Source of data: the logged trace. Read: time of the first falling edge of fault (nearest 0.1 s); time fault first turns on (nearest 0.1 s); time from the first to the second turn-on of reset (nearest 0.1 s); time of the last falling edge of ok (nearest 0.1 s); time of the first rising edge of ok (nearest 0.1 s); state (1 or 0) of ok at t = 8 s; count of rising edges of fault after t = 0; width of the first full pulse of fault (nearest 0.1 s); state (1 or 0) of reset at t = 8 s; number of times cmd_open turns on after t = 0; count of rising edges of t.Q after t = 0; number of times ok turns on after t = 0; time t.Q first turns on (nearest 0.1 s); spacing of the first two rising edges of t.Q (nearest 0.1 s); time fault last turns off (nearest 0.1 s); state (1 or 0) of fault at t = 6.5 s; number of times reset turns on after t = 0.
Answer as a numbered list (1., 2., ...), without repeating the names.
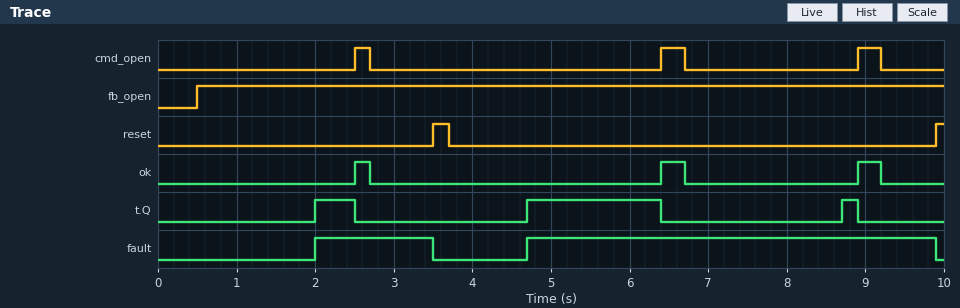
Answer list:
1. 3.5 s
2. 2.0 s
3. 6.4 s
4. 9.2 s
5. 2.5 s
6. 0
7. 2
8. 1.5 s
9. 0
10. 3
11. 3
12. 3
13. 2.0 s
14. 2.7 s
15. 9.9 s
16. 1
17. 2
